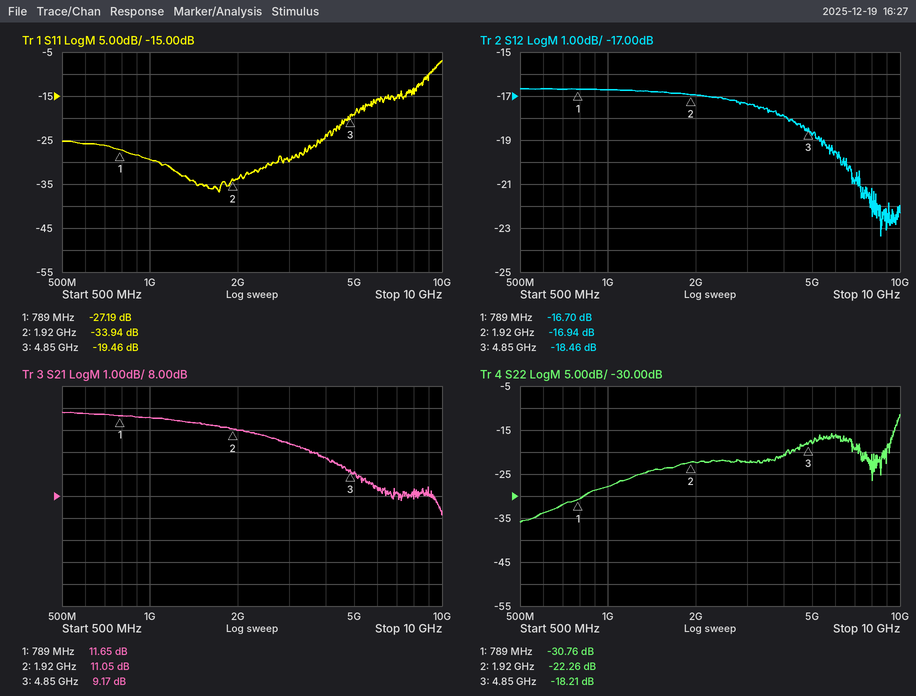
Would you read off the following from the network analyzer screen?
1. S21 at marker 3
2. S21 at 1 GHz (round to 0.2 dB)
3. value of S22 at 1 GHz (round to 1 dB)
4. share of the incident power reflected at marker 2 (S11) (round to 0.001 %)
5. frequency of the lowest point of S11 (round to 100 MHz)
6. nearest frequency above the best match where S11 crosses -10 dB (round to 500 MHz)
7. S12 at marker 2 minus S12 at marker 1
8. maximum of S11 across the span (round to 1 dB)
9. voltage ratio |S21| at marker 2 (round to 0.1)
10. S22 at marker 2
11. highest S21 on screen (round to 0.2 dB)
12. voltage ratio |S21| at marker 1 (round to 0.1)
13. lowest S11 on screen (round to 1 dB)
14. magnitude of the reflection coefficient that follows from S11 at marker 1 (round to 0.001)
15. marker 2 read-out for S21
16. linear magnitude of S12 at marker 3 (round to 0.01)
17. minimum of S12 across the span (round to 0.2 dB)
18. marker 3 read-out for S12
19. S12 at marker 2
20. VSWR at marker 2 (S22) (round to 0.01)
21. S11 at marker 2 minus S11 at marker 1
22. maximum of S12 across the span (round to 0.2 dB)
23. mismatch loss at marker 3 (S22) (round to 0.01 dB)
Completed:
9.17 dB
11.6 dB
-28 dB
0.040 %
1.7 GHz
9.0 GHz
-0.24 dB
-7 dB
3.6
-22.26 dB
11.8 dB
3.8
-37 dB
0.044
11.05 dB
0.12
-23.4 dB
-18.46 dB
-16.94 dB
1.17
-6.75 dB
-16.6 dB
0.07 dB
